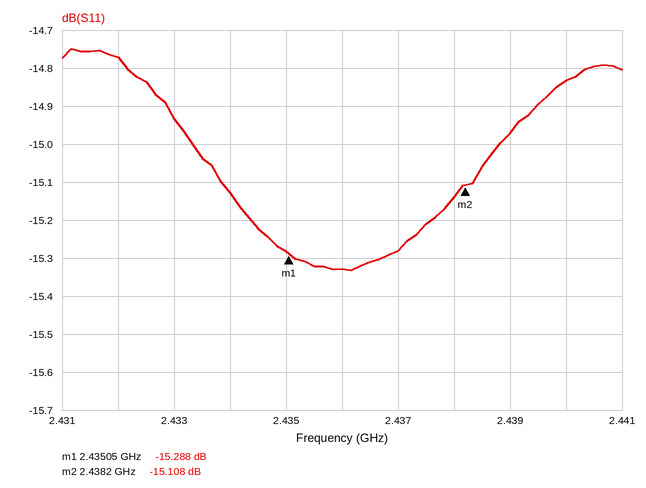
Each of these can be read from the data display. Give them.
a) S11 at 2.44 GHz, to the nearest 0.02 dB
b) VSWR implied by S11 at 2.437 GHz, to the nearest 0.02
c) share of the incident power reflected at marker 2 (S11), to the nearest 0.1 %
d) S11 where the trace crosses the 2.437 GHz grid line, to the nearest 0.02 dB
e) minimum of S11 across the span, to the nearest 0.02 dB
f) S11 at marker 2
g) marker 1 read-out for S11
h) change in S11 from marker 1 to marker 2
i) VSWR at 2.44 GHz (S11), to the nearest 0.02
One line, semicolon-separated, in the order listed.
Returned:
-14.84 dB; 1.42; 3.1 %; -15.28 dB; -15.34 dB; -15.108 dB; -15.288 dB; 0.180 dB; 1.44
